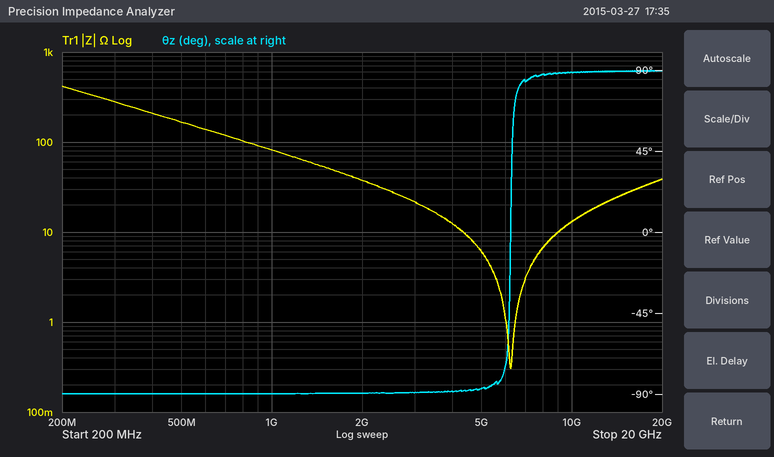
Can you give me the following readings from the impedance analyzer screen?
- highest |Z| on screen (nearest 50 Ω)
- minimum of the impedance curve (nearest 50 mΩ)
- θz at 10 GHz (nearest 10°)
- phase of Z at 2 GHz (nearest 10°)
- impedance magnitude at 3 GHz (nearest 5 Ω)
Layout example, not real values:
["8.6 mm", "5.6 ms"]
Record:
["400 Ω", "300 mΩ", "90°", "-90°", "20 Ω"]
